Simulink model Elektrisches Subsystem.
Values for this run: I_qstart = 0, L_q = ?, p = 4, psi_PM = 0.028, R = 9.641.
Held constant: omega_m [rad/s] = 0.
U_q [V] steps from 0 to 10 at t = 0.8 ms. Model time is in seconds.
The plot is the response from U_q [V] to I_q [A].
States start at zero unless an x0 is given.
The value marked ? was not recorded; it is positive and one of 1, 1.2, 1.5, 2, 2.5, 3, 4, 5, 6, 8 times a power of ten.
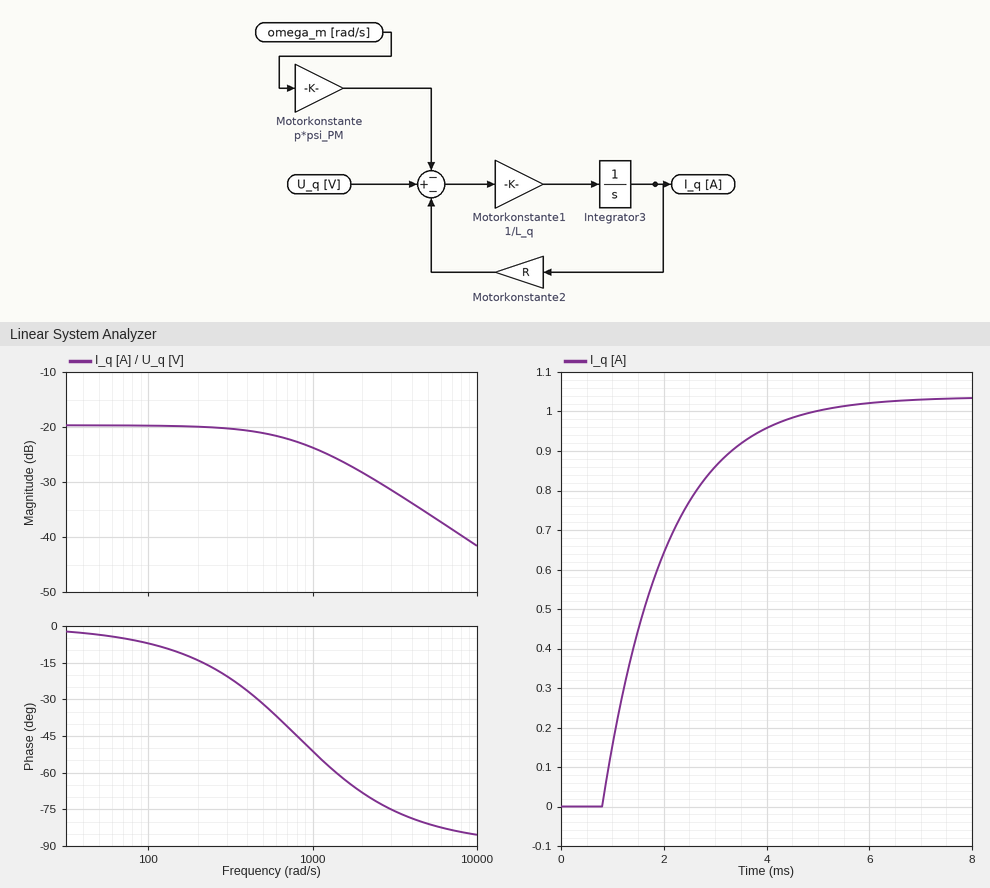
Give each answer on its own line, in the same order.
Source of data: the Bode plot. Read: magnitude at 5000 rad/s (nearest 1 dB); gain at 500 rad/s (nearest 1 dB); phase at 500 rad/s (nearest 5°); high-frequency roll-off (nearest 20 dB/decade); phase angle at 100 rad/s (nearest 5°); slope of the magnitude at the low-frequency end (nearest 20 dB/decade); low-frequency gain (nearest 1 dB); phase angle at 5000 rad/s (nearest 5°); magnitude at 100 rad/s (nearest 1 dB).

-36 dB
-21 dB
-30°
-20 dB/decade
-5°
0 dB/decade
-20 dB
-80°
-20 dB
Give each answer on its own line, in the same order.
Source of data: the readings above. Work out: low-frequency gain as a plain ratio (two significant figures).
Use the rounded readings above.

0.10
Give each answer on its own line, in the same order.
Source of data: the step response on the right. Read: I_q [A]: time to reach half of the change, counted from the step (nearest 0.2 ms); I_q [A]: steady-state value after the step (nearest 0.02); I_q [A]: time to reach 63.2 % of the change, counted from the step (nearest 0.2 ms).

0.8 ms
1.04
1.2 ms
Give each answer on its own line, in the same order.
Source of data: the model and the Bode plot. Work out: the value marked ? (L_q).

0.012
